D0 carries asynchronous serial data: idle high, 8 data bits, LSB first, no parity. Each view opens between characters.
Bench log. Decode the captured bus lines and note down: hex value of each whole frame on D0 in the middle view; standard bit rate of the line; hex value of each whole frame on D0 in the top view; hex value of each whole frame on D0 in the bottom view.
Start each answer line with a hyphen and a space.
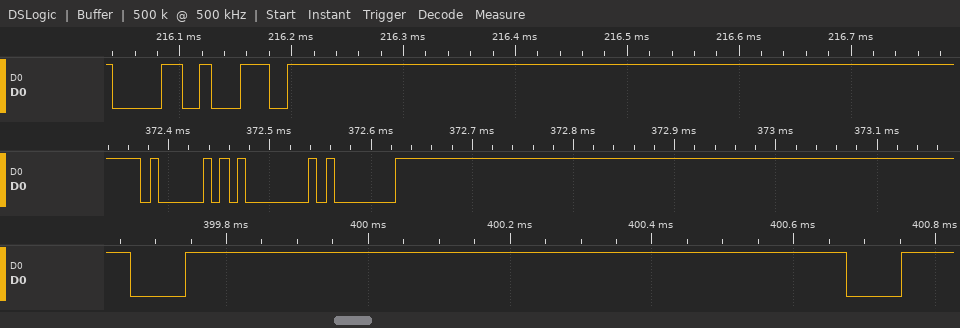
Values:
- 41, 01, 01
- 115200 baud
- 30, 9C
- 00, 00
